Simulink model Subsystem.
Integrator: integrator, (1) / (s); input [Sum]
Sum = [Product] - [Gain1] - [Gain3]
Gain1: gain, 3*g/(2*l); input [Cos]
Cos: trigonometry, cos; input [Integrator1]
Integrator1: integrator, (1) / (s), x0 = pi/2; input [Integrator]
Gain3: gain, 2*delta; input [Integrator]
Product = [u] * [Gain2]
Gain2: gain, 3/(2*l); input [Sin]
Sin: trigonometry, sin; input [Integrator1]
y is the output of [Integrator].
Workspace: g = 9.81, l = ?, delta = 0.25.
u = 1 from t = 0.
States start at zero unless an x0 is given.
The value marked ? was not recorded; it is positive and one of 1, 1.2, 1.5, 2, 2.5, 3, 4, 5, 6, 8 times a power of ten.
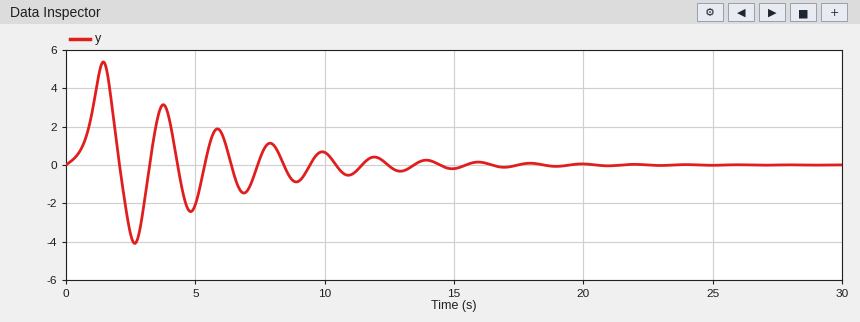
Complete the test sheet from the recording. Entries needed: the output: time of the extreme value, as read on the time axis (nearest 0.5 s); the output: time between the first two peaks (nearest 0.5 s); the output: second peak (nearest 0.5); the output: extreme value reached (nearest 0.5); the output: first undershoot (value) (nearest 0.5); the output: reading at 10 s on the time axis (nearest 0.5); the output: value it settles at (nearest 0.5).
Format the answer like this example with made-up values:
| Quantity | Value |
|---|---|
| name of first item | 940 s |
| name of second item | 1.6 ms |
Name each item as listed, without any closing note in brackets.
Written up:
| Quantity | Value |
|---|---|
| the output: time of the extreme value, as read on the time axis | 1.5 s |
| the output: time between the first two peaks | 2.5 s |
| the output: second peak | 3.0 |
| the output: extreme value reached | 5.5 |
| the output: first undershoot (value) | -4.0 |
| the output: reading at 10 s on the time axis | 0.5 |
| the output: value it settles at | 0.0 |
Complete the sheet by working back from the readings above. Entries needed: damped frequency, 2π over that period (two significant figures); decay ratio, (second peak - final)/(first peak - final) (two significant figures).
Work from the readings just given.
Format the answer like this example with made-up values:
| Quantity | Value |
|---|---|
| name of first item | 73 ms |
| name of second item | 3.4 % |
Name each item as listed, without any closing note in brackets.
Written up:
| Quantity | Value |
|---|---|
| damped frequency, 2π over that period | 2.5 rad/s |
| decay ratio, (second peak - final)/(first peak - final) | 0.55 |
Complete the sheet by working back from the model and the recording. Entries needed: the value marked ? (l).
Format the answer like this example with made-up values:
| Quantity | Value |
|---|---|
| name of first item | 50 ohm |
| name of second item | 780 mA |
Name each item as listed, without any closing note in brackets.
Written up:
| Quantity | Value |
|---|---|
| the value marked ? | 1.5 |
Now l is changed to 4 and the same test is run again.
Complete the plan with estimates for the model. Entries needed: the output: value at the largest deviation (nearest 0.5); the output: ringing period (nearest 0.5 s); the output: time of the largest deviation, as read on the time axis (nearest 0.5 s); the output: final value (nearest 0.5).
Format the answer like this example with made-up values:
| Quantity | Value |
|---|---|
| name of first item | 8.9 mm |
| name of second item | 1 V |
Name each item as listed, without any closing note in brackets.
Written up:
| Quantity | Value |
|---|---|
| the output: value at the largest deviation | 3.0 |
| the output: ringing period | 3.5 s |
| the output: time of the largest deviation, as read on the time axis | 2.5 s |
| the output: final value | 0.0 |
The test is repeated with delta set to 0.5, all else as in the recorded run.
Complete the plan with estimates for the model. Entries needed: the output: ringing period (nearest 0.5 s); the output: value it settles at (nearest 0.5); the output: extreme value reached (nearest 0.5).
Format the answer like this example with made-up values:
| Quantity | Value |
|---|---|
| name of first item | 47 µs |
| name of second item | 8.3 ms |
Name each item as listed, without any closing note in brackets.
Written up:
| Quantity | Value |
|---|---|
| the output: ringing period | 2.0 s |
| the output: value it settles at | 0.0 |
| the output: extreme value reached | 4.5 |
